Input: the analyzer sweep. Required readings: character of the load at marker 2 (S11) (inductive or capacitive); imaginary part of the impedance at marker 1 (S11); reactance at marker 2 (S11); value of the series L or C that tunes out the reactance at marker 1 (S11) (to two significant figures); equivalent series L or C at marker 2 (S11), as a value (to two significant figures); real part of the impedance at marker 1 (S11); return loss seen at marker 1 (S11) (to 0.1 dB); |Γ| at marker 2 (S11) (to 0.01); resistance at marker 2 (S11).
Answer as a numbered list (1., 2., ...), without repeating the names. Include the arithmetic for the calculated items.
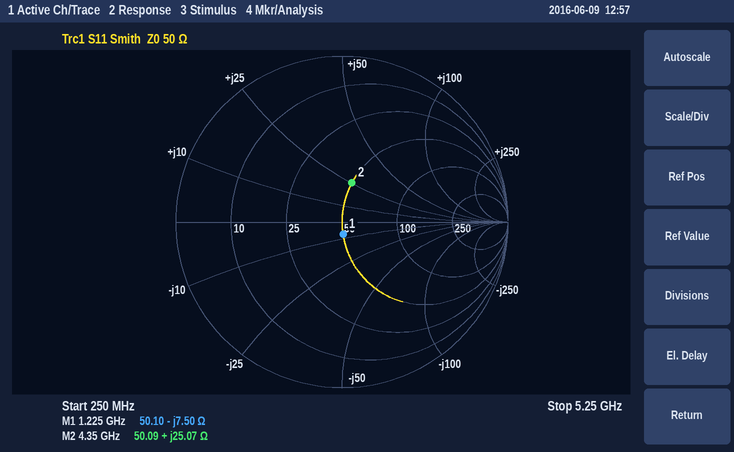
1. inductive
2. -7.50 Ω
3. +25.07 Ω
4. L = 7.5 Ω/(2π × 1.225 GHz) ≈ 974 pH, so 970 pH to two significant figures
5. L = 25.07 Ω/(2π × 4.35 GHz) ≈ 917 pH, so 920 pH to two significant figures
6. 50.10 Ω
7. 22.5 dB
8. 0.24
9. 50.09 Ω
